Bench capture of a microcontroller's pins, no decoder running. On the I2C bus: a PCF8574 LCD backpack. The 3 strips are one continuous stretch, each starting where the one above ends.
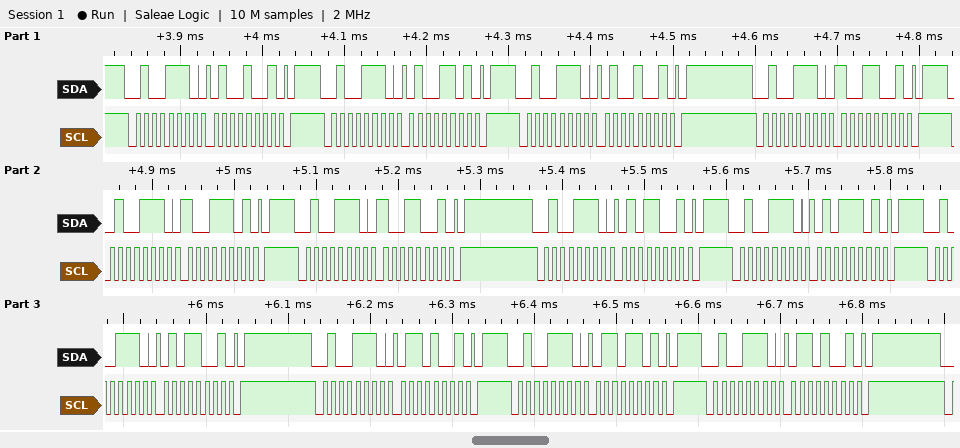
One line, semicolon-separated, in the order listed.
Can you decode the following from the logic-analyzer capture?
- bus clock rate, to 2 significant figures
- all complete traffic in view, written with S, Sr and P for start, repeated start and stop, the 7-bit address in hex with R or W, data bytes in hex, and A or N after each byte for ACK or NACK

100 kHz; S 27W A 49 A P S 27W A 4D A P S 27W A 49 A P S 27W A 99 A P S 27W A 9D A P S 27W A 99 A P S 27W A 59 A P S 27W A 5D A P S 27W A 59 A P S 27W A 69 A P S 27W A 6D A P S 27W A 69 A P
